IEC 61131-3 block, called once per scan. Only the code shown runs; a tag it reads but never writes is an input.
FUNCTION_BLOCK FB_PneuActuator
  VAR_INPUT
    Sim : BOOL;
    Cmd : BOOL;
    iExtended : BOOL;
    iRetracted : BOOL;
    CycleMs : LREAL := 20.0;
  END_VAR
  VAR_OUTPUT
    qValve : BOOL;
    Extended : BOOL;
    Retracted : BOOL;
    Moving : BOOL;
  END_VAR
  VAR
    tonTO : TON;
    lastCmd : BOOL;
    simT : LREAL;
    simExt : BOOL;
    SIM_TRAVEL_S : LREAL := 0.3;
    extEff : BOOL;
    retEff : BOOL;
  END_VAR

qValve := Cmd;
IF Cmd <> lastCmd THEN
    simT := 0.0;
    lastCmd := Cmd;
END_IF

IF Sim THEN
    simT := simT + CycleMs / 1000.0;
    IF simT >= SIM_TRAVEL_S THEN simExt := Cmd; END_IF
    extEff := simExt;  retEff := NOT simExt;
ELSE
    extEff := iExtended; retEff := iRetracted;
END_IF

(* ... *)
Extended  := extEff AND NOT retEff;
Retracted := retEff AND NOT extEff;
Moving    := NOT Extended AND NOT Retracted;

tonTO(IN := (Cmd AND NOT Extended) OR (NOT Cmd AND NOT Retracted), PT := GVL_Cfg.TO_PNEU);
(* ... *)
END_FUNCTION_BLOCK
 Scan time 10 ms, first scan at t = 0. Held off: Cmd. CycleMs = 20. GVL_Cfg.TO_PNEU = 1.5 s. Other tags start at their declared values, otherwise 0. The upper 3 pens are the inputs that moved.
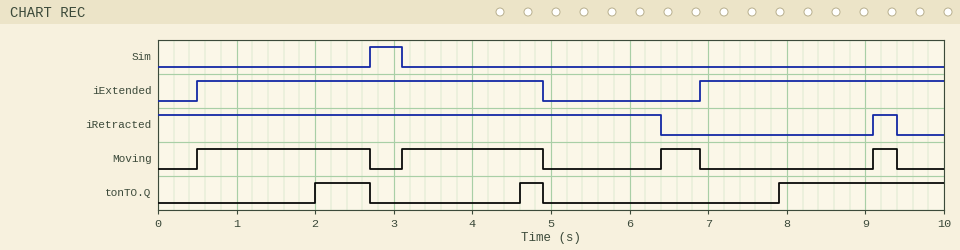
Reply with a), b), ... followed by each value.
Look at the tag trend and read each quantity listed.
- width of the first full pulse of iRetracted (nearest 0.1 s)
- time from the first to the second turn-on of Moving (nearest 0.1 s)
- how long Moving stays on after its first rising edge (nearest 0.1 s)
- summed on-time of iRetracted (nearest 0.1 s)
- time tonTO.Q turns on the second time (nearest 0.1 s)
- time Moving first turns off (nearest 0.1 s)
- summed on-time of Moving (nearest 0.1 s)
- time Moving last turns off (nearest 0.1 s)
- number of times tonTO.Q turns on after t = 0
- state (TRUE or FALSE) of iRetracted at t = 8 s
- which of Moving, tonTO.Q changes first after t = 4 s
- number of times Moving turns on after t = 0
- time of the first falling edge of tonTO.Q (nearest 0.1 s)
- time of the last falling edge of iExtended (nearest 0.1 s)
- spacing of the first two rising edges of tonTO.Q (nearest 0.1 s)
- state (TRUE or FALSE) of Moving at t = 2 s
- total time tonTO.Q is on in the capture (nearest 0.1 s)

a) 0.3 s
b) 2.6 s
c) 2.2 s
d) 6.7 s
e) 4.6 s
f) 2.7 s
g) 4.8 s
h) 9.4 s
i) 3
j) FALSE
k) tonTO.Q
l) 4
m) 2.7 s
n) 4.9 s
o) 2.6 s
p) TRUE
q) 3.1 s
